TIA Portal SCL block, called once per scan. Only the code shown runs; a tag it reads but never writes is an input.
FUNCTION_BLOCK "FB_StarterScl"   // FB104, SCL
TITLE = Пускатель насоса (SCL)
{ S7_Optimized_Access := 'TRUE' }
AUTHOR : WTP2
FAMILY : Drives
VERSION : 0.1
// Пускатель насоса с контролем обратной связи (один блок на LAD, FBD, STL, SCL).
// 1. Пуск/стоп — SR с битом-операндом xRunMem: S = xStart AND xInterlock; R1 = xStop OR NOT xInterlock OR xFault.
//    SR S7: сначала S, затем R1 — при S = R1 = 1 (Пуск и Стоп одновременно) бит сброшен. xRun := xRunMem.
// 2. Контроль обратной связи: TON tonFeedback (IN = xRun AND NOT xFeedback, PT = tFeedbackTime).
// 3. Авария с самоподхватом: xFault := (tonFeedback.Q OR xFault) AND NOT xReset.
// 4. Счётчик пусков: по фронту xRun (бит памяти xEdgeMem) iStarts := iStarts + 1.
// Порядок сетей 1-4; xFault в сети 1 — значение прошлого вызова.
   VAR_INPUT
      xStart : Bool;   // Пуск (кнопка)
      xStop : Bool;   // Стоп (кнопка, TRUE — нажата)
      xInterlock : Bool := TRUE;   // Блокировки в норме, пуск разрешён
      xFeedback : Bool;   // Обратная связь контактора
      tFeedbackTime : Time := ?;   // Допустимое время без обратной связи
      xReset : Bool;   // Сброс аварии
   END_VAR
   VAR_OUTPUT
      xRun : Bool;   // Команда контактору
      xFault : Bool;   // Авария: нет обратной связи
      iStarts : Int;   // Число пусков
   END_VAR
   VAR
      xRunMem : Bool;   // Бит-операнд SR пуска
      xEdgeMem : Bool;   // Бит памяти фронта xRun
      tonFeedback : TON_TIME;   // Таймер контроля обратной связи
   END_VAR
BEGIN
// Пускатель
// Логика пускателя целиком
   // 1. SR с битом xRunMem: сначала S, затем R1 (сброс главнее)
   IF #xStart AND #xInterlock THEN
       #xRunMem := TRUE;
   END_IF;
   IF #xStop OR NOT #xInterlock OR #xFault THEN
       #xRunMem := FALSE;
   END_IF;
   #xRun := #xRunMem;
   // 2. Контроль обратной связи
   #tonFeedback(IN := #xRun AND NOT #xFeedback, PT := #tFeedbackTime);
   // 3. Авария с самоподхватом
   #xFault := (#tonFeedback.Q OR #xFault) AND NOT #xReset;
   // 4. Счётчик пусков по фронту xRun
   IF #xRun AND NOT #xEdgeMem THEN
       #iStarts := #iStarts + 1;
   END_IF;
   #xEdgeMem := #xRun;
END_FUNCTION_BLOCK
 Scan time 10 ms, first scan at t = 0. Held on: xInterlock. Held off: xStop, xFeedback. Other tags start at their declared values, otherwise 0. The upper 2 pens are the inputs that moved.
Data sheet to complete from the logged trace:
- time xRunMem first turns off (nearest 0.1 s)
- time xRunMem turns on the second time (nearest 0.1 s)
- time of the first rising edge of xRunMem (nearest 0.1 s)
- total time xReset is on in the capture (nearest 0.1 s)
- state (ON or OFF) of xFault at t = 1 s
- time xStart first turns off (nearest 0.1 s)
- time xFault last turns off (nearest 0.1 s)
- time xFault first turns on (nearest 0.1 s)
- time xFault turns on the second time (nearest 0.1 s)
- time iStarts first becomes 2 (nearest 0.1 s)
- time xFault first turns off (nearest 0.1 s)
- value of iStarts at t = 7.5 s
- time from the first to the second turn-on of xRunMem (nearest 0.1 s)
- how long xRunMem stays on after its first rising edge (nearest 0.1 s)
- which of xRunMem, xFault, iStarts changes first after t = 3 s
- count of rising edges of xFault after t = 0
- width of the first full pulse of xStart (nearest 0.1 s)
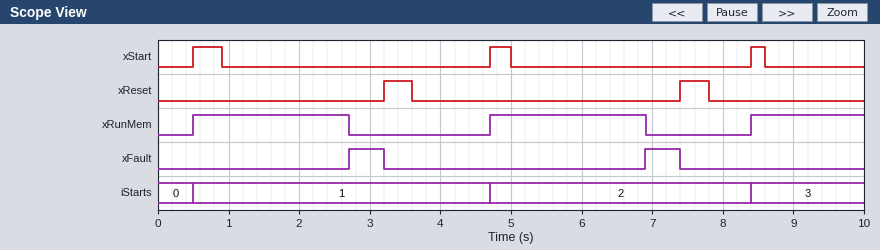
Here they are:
2.7 s
4.7 s
0.5 s
0.8 s
OFF
0.9 s
7.4 s
2.7 s
6.9 s
4.7 s
3.2 s
2
4.2 s
2.2 s
xFault
2
0.4 s
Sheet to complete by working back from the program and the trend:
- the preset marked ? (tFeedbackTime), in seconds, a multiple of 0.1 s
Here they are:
2.2 s
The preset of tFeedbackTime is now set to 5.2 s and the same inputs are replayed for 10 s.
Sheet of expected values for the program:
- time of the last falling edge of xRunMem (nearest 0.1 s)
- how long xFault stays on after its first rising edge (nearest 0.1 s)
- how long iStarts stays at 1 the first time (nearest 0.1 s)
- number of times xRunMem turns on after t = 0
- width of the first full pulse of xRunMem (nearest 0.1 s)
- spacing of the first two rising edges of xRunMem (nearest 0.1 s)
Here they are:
5.7 s
1.7 s
7.9 s
2
5.2 s
7.9 s
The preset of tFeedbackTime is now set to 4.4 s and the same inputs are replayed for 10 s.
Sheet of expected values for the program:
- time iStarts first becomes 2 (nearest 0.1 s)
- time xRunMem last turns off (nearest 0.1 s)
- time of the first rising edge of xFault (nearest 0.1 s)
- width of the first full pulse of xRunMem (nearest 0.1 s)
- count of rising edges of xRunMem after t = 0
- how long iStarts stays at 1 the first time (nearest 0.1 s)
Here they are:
8.4 s
4.9 s
4.9 s
4.4 s
2
7.9 s
